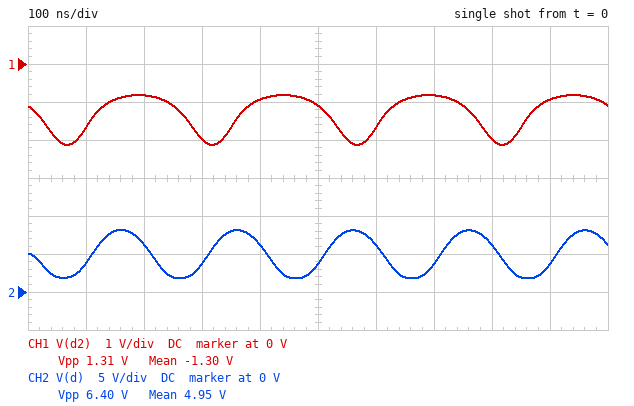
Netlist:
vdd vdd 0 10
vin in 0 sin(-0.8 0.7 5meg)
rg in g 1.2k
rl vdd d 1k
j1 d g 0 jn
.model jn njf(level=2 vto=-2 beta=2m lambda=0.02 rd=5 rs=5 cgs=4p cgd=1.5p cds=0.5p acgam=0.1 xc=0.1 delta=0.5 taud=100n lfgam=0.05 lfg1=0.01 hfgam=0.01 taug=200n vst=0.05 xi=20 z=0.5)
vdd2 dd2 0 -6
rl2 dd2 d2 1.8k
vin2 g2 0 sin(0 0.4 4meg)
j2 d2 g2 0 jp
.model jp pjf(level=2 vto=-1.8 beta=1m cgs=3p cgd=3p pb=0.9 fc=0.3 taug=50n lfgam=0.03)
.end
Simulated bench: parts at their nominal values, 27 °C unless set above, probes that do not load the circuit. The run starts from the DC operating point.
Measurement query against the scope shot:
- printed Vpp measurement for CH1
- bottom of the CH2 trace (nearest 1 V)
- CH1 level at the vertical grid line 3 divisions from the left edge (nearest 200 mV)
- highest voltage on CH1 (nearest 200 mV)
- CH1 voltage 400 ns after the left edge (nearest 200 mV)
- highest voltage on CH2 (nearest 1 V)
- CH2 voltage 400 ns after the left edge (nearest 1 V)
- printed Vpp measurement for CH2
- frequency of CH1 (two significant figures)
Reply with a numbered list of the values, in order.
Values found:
1. 1.31 V
2. 2 V
3. -2.0 V
4. -800 mV
5. -1.0 V
6. 8 V
7. 6 V
8. 6.40 V
9. 4.0 MHz
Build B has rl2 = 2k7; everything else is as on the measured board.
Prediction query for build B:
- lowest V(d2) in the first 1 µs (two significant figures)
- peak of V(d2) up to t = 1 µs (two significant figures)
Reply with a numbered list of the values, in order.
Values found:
1. -1.1 V
2. -530 mV
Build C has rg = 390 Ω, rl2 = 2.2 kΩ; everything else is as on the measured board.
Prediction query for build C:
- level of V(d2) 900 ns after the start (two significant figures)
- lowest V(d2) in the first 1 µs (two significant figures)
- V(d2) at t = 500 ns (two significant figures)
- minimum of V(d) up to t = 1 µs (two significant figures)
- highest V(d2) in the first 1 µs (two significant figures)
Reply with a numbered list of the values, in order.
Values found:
1. -740 mV
2. -1.5 V
3. -850 mV
4. 1.7 V
5. -660 mV
